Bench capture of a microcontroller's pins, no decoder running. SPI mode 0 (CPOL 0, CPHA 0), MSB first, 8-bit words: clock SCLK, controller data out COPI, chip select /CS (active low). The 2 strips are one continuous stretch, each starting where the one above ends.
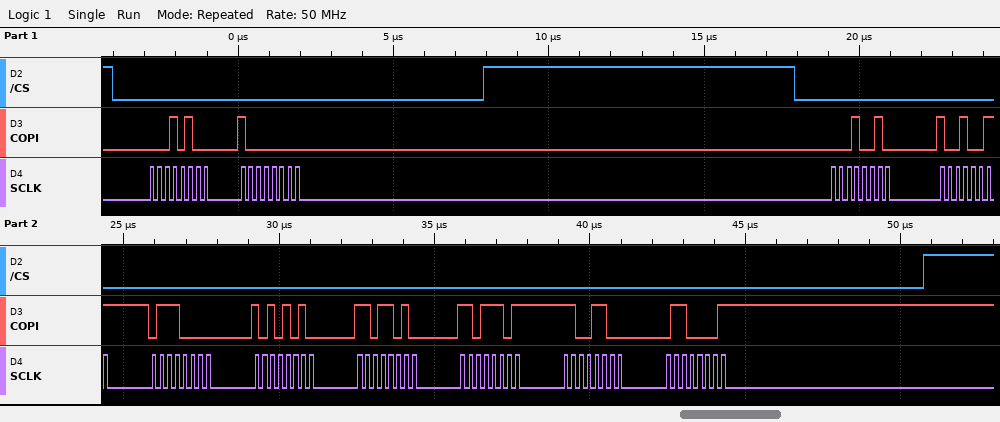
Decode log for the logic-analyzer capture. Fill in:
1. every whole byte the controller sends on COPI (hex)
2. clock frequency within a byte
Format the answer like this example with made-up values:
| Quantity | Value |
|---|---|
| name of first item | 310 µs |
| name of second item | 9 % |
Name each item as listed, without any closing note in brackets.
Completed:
| Quantity | Value |
|---|---|
| every whole byte the controller sends on COPI | 14 80 12 93 70 AA DA DD CC 61 |
| clock frequency within a byte | 4 MHz |
